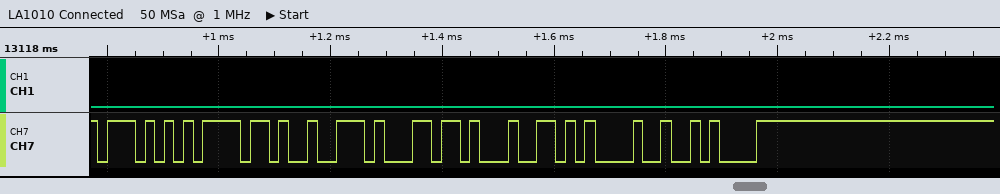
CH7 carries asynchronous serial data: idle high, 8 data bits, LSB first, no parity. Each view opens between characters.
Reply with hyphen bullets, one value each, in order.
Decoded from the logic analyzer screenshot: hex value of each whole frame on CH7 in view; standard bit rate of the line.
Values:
- 57, 6F, 72, 6C, 64, 21, 0A
- 57600 baud
